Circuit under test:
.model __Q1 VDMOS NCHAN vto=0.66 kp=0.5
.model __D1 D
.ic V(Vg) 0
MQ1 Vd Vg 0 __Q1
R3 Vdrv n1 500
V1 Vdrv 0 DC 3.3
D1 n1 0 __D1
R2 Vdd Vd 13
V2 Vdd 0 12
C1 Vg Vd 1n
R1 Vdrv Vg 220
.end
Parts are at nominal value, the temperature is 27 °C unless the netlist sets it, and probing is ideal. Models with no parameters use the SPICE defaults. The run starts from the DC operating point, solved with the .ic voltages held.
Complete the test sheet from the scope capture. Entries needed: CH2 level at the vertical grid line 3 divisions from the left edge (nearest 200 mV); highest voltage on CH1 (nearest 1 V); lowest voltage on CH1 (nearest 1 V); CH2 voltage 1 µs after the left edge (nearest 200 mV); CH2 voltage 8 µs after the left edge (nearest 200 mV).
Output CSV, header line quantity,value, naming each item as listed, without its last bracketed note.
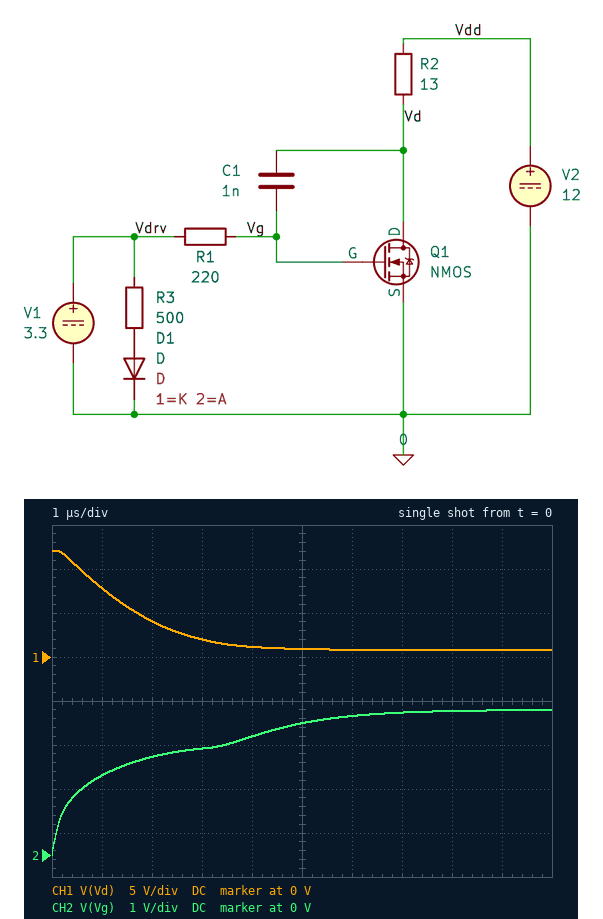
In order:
quantity,value
CH2 level at the vertical grid line 3 divisions from the left edge,2.4 V
highest voltage on CH1,12 V
lowest voltage on CH1,1 V
CH2 voltage 1 µs after the left edge,1.8 V
CH2 voltage 8 µs after the left edge,3.2 V
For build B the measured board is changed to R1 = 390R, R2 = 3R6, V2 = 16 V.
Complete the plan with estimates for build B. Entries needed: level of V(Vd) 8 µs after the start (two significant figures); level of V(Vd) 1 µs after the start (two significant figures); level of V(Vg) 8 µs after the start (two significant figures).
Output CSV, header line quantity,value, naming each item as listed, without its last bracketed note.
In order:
quantity,value
level of V(Vd) 8 µs after the start,10 V
level of V(Vd) 1 µs after the start,15 V
level of V(Vg) 8 µs after the start,3.2 V
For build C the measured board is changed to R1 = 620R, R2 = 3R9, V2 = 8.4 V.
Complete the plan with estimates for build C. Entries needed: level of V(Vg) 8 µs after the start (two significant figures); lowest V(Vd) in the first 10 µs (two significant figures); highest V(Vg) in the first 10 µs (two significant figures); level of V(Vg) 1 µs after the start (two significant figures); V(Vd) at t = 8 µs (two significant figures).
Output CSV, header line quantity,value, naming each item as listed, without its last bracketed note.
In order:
quantity,value
level of V(Vg) 8 µs after the start,2.9 V
lowest V(Vd) in the first 10 µs,3.1 V
highest V(Vg) in the first 10 µs,3.0 V
level of V(Vg) 1 µs after the start,1.4 V
V(Vd) at t = 8 µs,3.5 V
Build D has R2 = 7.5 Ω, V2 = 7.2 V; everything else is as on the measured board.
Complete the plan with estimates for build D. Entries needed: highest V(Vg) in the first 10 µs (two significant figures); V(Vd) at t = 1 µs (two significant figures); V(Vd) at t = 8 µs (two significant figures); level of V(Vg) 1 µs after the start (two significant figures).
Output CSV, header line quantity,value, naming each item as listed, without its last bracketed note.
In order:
quantity,value
highest V(Vg) in the first 10 µs,3.3 V
V(Vd) at t = 1 µs,4.1 V
V(Vd) at t = 8 µs,760 mV
level of V(Vg) 1 µs after the start,2.0 V
